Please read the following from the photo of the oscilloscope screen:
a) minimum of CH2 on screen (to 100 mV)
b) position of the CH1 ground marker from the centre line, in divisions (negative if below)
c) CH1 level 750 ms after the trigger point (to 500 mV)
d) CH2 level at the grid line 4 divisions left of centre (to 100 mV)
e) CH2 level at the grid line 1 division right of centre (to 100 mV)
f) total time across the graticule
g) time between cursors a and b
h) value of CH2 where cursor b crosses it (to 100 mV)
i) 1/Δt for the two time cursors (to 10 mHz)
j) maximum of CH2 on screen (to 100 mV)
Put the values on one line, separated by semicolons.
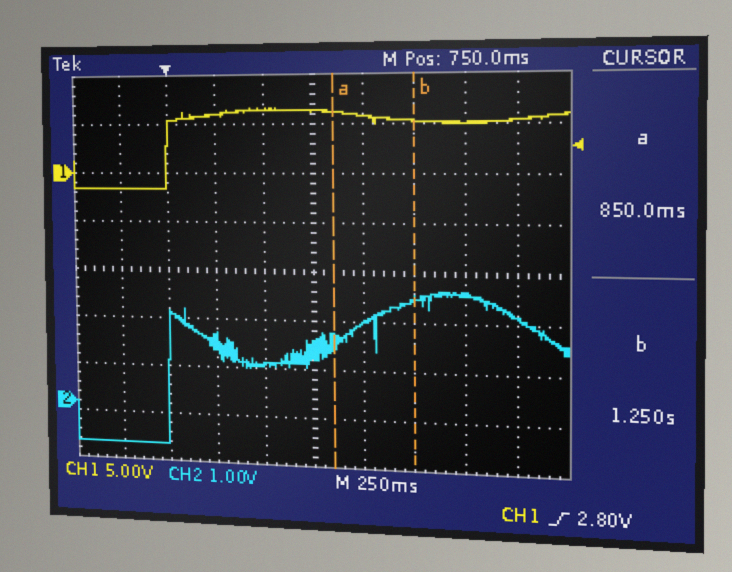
-800 mV; +2.0 div; 6.5 V; -800 mV; 1.8 V; 2.5 s; 400 ms; 2.3 V; 2.50 Hz; 2.4 V
